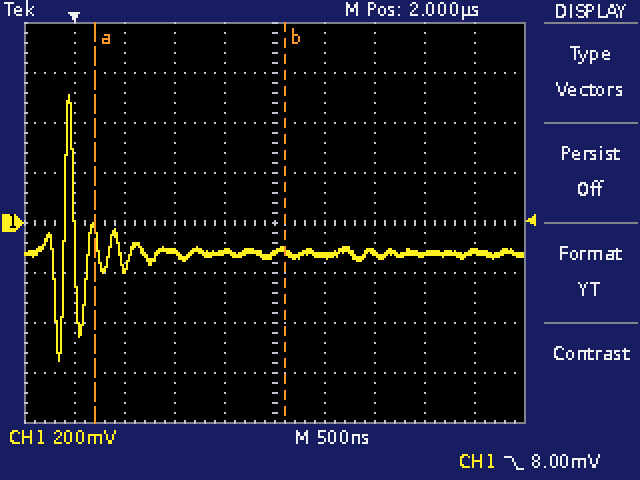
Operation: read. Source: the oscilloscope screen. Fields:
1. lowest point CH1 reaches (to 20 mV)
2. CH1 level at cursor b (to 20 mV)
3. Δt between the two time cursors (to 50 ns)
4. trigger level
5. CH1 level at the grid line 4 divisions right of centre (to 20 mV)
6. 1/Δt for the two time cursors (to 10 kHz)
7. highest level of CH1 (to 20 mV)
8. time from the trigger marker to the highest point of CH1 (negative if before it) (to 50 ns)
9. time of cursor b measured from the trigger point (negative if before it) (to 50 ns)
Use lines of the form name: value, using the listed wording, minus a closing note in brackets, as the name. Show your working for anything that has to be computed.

lowest point CH1 reaches: -560 mV
CH1 level at cursor b: -120 mV
Δt between the two time cursors: 1.90 µs
trigger level: 8.00 mV
CH1 level at the grid line 4 divisions right of centre: -120 mV
1/Δt for the two time cursors: 1 / 1.90 µs ≈ 530 kHz
highest level of CH1: 520 mV
time from the trigger marker to the highest point of CH1 (negative if before it): -50 ns
time of cursor b measured from the trigger point (negative if before it): +2.10 µs
